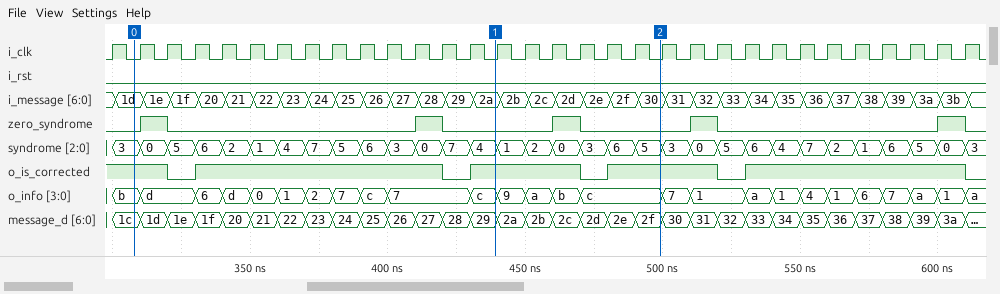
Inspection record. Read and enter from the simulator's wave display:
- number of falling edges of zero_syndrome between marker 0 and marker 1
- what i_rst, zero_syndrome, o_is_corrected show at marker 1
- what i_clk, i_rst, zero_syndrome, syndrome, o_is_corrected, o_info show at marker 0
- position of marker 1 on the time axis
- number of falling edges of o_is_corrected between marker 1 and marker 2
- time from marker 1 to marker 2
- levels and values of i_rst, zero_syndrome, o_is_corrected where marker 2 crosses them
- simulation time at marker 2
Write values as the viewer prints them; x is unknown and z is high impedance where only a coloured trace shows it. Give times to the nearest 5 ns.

2
i_rst=0, zero_syndrome=0, o_is_corrected=1
i_clk=0, i_rst=0, zero_syndrome=0, syndrome=3, o_is_corrected=1, o_info=b
440 ns
1
60 ns
i_rst=0, zero_syndrome=0, o_is_corrected=1
500 ns
